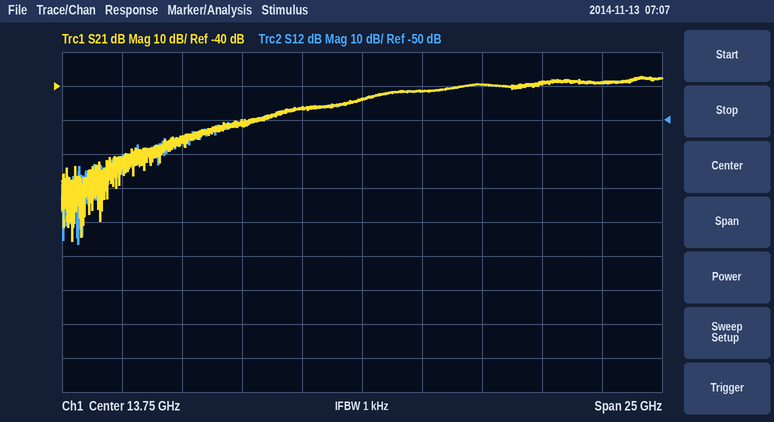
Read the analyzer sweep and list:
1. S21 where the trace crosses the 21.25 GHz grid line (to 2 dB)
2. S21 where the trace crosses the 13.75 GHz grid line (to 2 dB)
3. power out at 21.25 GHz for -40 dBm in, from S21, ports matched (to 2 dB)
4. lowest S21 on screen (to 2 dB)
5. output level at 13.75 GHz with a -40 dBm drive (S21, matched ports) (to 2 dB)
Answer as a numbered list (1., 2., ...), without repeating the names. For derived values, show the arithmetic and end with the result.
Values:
1. -40 dB
2. -44 dB
3. -40 dBm + (-40 dB) = -80 dBm
4. -86 dB
5. -40 dBm + (-44 dB) = -84 dBm
